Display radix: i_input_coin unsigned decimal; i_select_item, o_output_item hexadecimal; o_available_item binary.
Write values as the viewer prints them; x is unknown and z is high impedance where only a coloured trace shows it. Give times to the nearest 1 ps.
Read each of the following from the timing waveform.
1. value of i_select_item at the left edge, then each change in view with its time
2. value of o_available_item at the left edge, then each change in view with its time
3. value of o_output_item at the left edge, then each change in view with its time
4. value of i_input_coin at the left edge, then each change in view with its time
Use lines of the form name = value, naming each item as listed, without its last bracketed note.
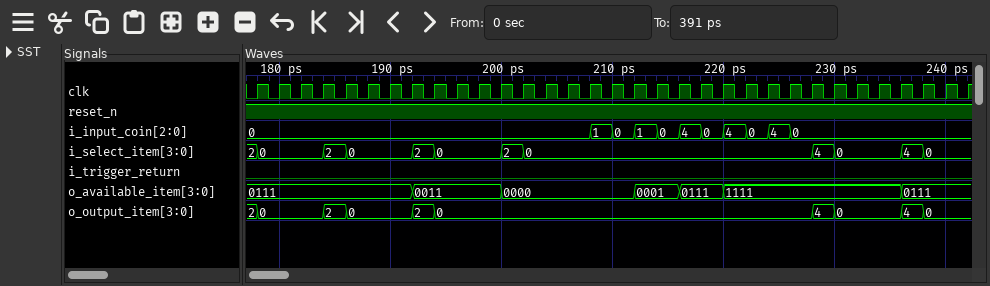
value of i_select_item at the left edge, then each change in view with its time = 2, 0 at 178 ps, 2 at 184 ps, 0 at 186 ps, 2 at 192 ps, 0 at 194 ps, 2 at 200 ps, 0 at 202 ps, 4 at 228 ps, 0 at 230 ps, 4 at 236 ps, 0 at 238 ps
value of o_available_item at the left edge, then each change in view with its time = 0111, 0011 at 192 ps, 0000 at 200 ps, 0001 at 212 ps, 0111 at 216 ps, 1111 at 220 ps, 0111 at 236 ps
value of o_output_item at the left edge, then each change in view with its time = 2, 0 at 178 ps, 2 at 184 ps, 0 at 186 ps, 2 at 192 ps, 0 at 194 ps, 4 at 228 ps, 0 at 230 ps, 4 at 236 ps, 0 at 238 ps
value of i_input_coin at the left edge, then each change in view with its time = 0, 1 at 208 ps, 0 at 210 ps, 1 at 212 ps, 0 at 214 ps, 4 at 216 ps, 0 at 218 ps, 4 at 220 ps, 0 at 222 ps, 4 at 224 ps, 0 at 226 ps
